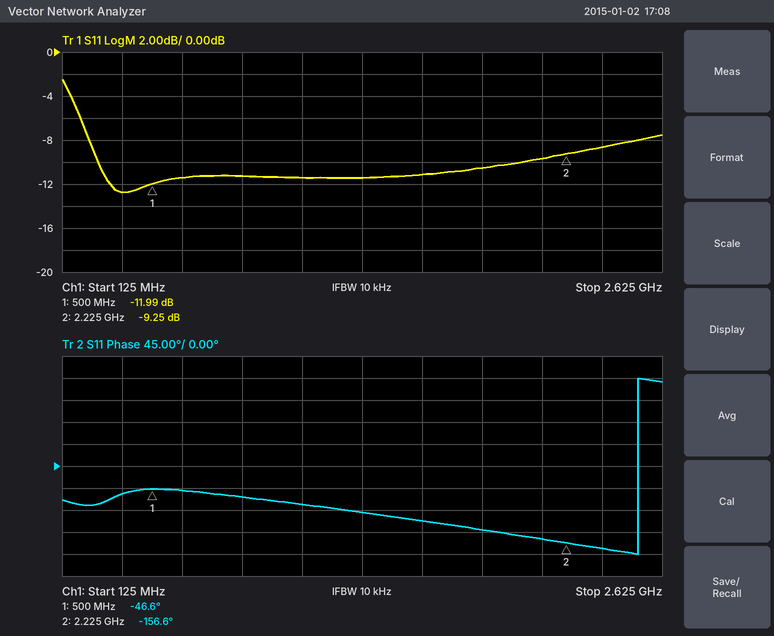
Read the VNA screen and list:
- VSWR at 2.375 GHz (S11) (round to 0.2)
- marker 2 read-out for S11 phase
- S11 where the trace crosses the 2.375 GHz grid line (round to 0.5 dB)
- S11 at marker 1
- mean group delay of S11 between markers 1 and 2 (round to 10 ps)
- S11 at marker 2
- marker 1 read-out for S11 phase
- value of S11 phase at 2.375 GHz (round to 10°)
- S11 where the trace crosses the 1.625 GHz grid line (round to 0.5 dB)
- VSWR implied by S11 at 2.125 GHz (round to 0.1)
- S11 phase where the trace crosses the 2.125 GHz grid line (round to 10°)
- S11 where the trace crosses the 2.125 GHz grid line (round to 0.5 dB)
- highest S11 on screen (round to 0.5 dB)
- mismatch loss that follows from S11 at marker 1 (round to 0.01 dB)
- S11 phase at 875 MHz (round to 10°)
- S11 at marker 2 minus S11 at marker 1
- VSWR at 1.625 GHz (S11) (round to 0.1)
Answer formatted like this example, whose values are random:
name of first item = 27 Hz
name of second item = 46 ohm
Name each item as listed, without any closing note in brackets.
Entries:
VSWR at 2.375 GHz (S11) = 2.2
marker 2 read-out for S11 phase = -156.6°
S11 where the trace crosses the 2.375 GHz grid line = -8.5 dB
S11 at marker 1 = -11.99 dB
mean group delay of S11 between markers 1 and 2 = 180 ps
S11 at marker 2 = -9.25 dB
marker 1 read-out for S11 phase = -46.6°
value of S11 phase at 2.375 GHz = -170°
S11 where the trace crosses the 1.625 GHz grid line = -11.0 dB
VSWR implied by S11 at 2.125 GHz = 2.0
S11 phase where the trace crosses the 2.125 GHz grid line = -150°
S11 where the trace crosses the 2.125 GHz grid line = -9.5 dB
highest S11 on screen = -2.5 dB
mismatch loss that follows from S11 at marker 1 = 0.28 dB
S11 phase at 875 MHz = -60°
S11 at marker 2 minus S11 at marker 1 = 2.74 dB
VSWR at 1.625 GHz (S11) = 1.8
